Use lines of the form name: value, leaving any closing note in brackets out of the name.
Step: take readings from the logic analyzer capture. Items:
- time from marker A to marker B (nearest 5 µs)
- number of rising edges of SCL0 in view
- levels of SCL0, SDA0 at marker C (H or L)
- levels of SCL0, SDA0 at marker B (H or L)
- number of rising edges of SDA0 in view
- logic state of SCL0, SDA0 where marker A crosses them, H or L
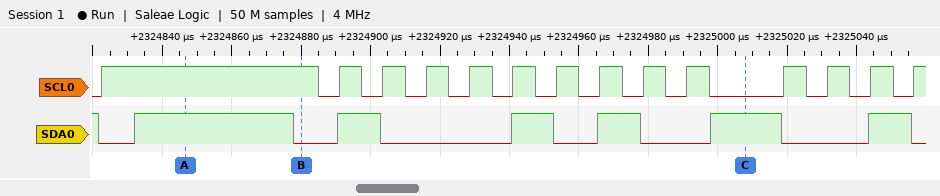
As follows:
time from marker A to marker B: 35 µs
number of rising edges of SCL0 in view: 14
levels of SCL0, SDA0 at marker C: SCL0=L, SDA0=H
levels of SCL0, SDA0 at marker B: SCL0=H, SDA0=L
number of rising edges of SDA0 in view: 6
logic state of SCL0, SDA0 where marker A crosses them, H or L: SCL0=H, SDA0=H
